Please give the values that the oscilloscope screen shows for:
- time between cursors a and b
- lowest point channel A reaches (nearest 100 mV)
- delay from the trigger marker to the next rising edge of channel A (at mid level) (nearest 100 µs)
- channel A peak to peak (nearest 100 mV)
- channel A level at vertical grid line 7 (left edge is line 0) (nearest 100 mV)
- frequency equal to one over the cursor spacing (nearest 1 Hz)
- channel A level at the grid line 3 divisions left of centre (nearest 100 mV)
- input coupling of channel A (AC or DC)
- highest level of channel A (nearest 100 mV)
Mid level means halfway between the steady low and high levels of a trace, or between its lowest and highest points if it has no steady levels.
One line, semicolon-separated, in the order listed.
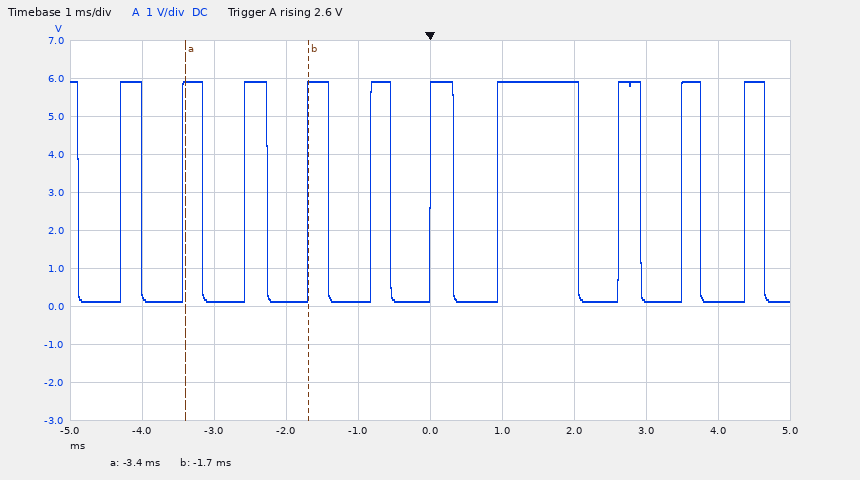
1.7 ms; 100 mV; 900 µs; 5.8 V; 5.9 V; 588 Hz; 100 mV; DC; 5.9 V
